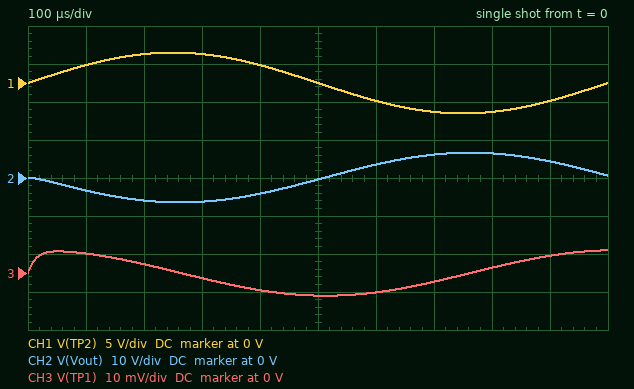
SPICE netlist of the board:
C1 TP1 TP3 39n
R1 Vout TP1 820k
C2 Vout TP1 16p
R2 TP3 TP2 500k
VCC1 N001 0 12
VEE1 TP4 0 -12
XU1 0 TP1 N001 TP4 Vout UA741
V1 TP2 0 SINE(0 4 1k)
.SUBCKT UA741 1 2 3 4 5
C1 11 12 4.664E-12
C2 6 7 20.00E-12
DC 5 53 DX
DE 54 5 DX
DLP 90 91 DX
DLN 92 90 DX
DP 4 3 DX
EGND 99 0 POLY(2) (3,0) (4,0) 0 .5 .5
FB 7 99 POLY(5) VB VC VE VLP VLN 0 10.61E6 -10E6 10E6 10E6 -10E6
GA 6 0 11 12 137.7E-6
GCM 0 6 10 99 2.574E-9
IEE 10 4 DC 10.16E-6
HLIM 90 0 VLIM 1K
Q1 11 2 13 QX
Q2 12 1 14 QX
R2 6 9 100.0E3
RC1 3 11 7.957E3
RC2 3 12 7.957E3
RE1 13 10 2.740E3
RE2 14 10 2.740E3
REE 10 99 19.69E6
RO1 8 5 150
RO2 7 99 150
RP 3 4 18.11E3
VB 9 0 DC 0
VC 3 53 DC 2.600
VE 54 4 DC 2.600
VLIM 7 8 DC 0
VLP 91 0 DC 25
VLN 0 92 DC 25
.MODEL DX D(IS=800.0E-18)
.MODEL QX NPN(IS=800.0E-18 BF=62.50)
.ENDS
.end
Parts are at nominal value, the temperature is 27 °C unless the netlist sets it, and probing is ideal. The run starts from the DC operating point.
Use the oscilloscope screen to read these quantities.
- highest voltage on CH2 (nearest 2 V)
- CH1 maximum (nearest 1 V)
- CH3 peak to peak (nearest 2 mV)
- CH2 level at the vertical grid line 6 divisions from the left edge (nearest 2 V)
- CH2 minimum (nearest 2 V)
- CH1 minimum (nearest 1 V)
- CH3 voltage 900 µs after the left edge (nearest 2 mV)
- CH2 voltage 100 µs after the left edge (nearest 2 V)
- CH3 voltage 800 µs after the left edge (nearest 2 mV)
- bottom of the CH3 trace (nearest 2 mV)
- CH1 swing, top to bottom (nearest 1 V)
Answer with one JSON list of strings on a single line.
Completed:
["6 V", "4 V", "12 mV", "4 V", "-6 V", "-4 V", "4 mV", "-4 V", "2 mV", "-6 mV", "8 V"]
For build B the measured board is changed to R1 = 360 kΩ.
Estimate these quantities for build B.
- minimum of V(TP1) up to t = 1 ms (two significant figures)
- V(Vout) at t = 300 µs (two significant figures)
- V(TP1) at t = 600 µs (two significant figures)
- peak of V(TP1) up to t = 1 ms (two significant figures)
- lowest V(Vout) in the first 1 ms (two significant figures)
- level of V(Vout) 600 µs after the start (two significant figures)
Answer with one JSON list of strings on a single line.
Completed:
["-2.6 mV", "-2.7 V", "-2.2 mV", "2.6 mV", "-2.8 V", "1.7 V"]
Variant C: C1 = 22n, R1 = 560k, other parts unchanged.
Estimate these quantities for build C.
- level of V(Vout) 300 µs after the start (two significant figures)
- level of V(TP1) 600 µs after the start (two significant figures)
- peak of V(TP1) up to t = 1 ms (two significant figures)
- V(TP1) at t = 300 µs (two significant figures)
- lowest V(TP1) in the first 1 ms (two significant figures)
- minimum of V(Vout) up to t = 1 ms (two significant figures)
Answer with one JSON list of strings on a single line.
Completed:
["-4.2 V", "-3.4 mV", "4.1 mV", "-1.1 mV", "-4.1 mV", "-4.4 V"]
